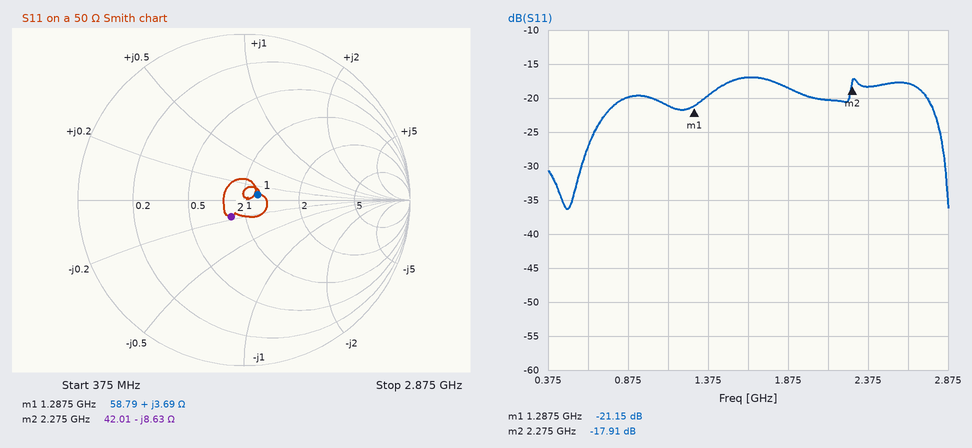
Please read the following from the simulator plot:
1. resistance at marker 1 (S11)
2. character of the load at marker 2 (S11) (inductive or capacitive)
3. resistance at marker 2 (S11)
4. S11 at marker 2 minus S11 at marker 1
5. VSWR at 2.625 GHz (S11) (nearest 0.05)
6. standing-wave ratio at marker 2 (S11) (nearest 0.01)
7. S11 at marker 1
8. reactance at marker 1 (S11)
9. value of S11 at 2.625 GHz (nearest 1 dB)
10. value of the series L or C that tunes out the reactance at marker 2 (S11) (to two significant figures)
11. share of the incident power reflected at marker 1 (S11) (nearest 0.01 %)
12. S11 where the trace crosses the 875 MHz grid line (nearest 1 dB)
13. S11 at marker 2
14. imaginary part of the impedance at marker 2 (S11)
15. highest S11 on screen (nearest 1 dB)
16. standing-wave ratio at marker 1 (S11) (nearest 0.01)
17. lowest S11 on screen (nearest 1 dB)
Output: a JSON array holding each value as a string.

["58.79 Ω", "capacitive", "42.01 Ω", "3.24 dB", "1.30", "1.29", "-21.15 dB", "+3.69 Ω", "-18 dB", "600 pH", "0.77 %", "-20 dB", "-17.91 dB", "-8.63 Ω", "-17 dB", "1.19", "-36 dB"]
